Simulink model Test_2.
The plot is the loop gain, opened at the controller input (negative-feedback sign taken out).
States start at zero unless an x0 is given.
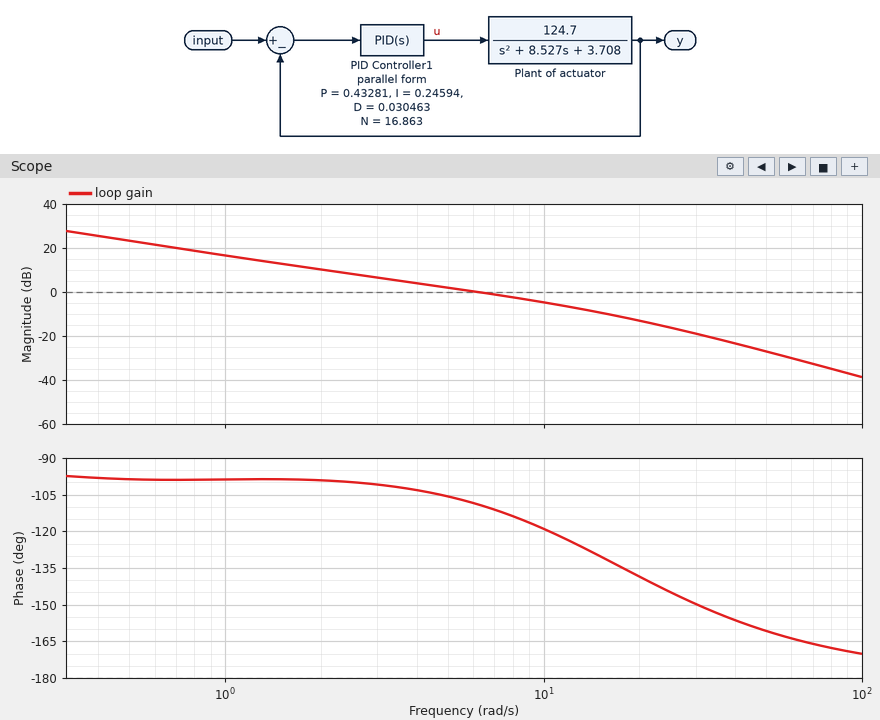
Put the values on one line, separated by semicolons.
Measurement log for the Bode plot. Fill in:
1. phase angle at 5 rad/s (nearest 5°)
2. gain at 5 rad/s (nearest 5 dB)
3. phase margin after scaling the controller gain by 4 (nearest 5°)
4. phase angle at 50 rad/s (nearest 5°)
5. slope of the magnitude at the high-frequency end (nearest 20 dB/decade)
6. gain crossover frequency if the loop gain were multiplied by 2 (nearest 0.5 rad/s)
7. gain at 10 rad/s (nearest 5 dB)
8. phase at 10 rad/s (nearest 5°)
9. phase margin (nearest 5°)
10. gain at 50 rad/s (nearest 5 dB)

-105°; 0 dB; 45°; -160°; -40 dB/decade; 11.5 rad/s; -5 dB; -120°; 70°; -25 dB
